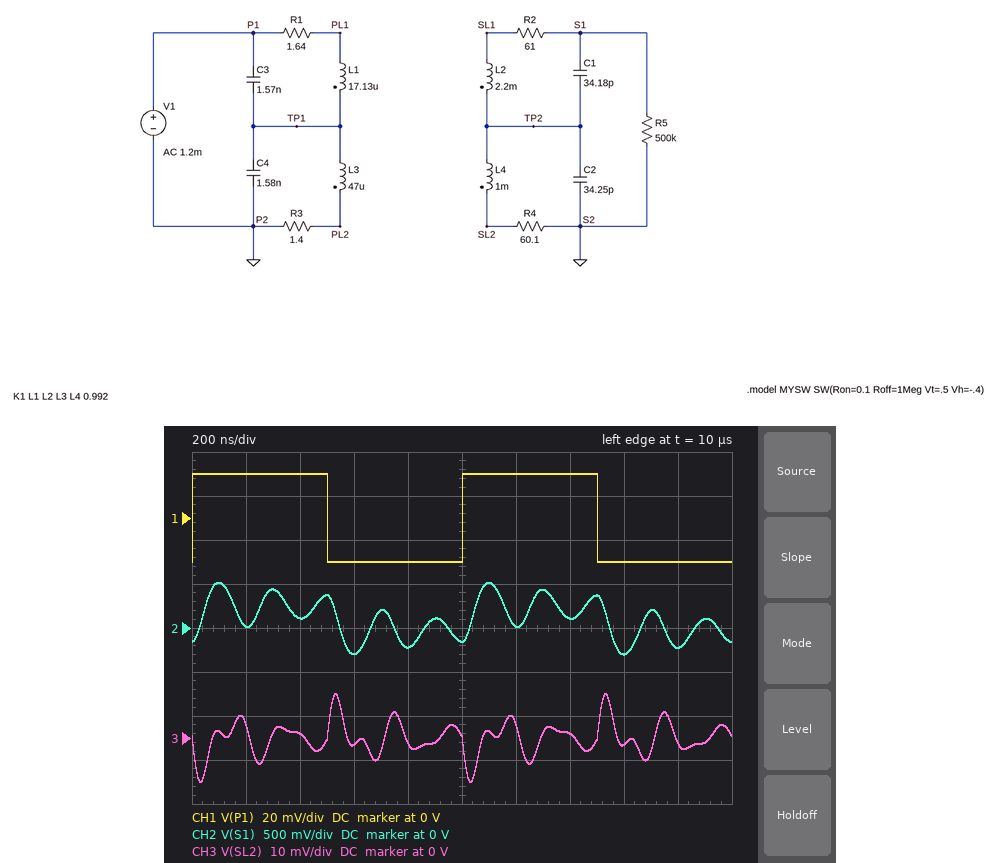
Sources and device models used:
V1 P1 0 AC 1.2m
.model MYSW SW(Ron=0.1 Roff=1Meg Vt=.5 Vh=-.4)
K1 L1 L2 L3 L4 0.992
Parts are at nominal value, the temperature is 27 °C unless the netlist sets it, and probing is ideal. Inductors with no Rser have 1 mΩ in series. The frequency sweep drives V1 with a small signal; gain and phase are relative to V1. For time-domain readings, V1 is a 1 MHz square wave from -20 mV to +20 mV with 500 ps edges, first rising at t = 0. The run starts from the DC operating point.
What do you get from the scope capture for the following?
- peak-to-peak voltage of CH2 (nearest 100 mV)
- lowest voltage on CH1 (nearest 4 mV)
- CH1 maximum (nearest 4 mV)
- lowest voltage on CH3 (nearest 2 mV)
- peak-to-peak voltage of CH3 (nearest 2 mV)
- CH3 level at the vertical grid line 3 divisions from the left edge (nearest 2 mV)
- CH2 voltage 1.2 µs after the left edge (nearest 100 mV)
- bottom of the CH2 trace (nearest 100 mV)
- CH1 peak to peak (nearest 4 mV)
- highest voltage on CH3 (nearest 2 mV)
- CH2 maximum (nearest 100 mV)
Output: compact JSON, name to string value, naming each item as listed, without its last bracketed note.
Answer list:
{"peak-to-peak voltage of CH2": "800 mV", "lowest voltage on CH1": "-20 mV", "CH1 maximum": "20 mV", "lowest voltage on CH3": "-10 mV", "peak-to-peak voltage of CH3": "20 mV", "CH3 level at the vertical grid line 3 divisions from the left edge": "-2 mV", "CH2 voltage 1.2 µs after the left edge": "0 V", "bottom of the CH2 trace": "-300 mV", "CH1 peak to peak": "40 mV", "highest voltage on CH3": "10 mV", "CH2 maximum": "500 mV"}
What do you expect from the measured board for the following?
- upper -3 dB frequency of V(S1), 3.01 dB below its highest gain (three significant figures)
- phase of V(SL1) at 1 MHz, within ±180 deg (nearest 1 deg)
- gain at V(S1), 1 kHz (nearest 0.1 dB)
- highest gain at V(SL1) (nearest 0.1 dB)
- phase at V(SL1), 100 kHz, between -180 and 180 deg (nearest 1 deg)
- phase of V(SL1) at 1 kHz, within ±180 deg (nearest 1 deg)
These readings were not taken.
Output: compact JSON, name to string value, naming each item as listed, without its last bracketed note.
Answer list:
{"upper -3 dB frequency of V(S1), 3.01 dB below its highest gain": "5.31 MHz", "phase of V(SL1) at 1 MHz, within ±180 deg": "-1 deg", "gain at V(S1), 1 kHz": "4.7 dB", "highest gain at V(SL1)": "32.7 dB", "phase at V(SL1), 100 kHz, between -180 and 180 deg": "2 deg", "phase of V(SL1) at 1 kHz, within ±180 deg": "76 deg"}
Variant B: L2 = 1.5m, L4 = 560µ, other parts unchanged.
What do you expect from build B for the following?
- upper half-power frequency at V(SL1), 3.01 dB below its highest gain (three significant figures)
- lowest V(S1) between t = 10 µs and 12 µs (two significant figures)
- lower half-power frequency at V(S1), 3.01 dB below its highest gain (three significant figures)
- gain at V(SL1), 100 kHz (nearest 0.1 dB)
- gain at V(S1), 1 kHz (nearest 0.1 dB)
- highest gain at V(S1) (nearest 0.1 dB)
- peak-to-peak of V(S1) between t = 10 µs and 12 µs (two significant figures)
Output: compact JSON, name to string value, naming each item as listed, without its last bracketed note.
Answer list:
{"upper half-power frequency at V(SL1), 3.01 dB below its highest gain": "6.43 MHz", "lowest V(S1) between t = 10 µs and 12 µs": "-120 mV", "lower half-power frequency at V(S1), 3.01 dB below its highest gain": "5.60 MHz", "gain at V(SL1), 100 kHz": "15.0 dB", "gain at V(S1), 1 kHz": "2.7 dB", "highest gain at V(S1)": "30.6 dB", "peak-to-peak of V(S1) between t = 10 µs and 12 µs": "420 mV"}
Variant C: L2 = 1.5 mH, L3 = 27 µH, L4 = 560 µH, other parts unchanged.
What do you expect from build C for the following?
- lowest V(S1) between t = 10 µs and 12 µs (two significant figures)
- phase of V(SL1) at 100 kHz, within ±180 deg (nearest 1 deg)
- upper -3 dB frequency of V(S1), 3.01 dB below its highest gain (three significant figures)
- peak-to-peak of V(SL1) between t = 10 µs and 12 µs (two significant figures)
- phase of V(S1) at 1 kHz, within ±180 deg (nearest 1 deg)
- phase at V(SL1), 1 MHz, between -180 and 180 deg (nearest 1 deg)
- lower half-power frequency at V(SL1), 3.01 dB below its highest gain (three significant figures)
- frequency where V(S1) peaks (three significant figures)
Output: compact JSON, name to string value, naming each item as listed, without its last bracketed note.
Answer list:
{"lowest V(S1) between t = 10 µs and 12 µs": "-170 mV", "phase of V(SL1) at 100 kHz, within ±180 deg": "3 deg", "upper -3 dB frequency of V(S1), 3.01 dB below its highest gain": "6.64 MHz", "peak-to-peak of V(SL1) between t = 10 µs and 12 µs": "530 mV", "phase of V(S1) at 1 kHz, within ±180 deg": "80 deg", "phase at V(SL1), 1 MHz, between -180 and 180 deg": "-1 deg", "lower half-power frequency at V(SL1), 3.01 dB below its highest gain": "5.58 MHz", "frequency where V(S1) peaks": "6.15 MHz"}
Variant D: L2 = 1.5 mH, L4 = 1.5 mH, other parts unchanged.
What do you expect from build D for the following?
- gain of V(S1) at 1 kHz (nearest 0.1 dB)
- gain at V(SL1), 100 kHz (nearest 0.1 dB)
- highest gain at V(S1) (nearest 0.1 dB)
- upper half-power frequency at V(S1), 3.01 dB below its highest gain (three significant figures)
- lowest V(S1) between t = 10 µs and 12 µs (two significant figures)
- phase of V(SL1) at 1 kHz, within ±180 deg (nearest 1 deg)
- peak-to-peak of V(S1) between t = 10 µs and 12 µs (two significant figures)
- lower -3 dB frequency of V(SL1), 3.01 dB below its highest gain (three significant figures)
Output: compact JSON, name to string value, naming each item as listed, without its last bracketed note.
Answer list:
{"gain of V(S1) at 1 kHz": "4.6 dB", "gain at V(SL1), 100 kHz": "16.9 dB", "highest gain at V(S1)": "32.8 dB", "upper half-power frequency at V(S1), 3.01 dB below its highest gain": "5.78 MHz", "lowest V(S1) between t = 10 µs and 12 µs": "-250 mV", "phase of V(SL1) at 1 kHz, within ±180 deg": "76 deg", "peak-to-peak of V(S1) between t = 10 µs and 12 µs": "720 mV", "lower -3 dB frequency of V(SL1), 3.01 dB below its highest gain": "4.96 MHz"}
